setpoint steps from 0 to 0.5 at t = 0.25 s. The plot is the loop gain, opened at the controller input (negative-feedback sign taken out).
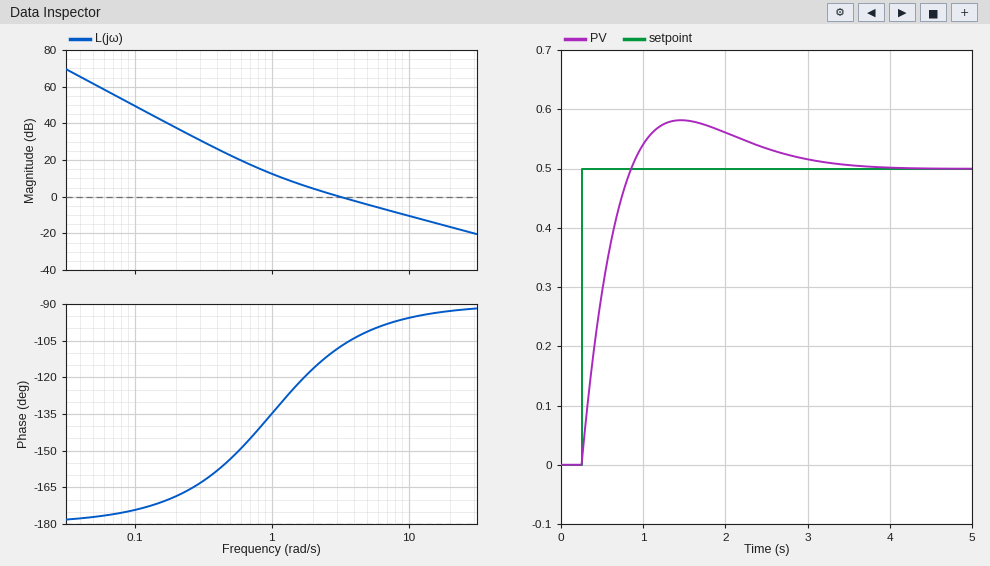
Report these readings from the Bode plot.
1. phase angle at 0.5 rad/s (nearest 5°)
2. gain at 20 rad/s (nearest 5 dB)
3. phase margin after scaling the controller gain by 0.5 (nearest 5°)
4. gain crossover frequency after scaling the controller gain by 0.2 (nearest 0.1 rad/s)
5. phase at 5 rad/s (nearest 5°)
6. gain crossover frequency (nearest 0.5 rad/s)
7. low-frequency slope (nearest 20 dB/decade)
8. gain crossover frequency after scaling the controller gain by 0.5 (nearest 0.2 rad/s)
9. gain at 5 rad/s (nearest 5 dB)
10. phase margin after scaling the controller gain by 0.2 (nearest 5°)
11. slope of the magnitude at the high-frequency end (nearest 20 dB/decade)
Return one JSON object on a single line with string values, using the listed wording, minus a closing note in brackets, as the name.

{"phase angle at 0.5 rad/s": "-155°", "gain at 20 rad/s": "-15 dB", "phase margin after scaling the controller gain by 0.5": "60°", "gain crossover frequency after scaling the controller gain by 0.2": "0.9 rad/s", "phase at 5 rad/s": "-100°", "gain crossover frequency": "3.0 rad/s", "low-frequency slope": "-40 dB/decade", "gain crossover frequency after scaling the controller gain by 0.5": "1.8 rad/s", "gain at 5 rad/s": "-5 dB", "phase margin after scaling the controller gain by 0.2": "40°", "slope of the magnitude at the high-frequency end": "-20 dB/decade"}
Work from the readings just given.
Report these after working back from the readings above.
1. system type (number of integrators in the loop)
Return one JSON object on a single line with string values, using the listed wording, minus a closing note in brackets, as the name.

{"system type": "2"}
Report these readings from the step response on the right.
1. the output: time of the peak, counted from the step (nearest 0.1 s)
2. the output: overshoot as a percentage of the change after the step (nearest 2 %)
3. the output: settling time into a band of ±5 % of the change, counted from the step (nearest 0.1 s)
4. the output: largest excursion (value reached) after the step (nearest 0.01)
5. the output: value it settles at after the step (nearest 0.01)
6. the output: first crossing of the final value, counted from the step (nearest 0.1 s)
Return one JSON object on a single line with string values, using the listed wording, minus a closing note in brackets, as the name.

{"the output: time of the peak, counted from the step": "1.2 s", "the output: overshoot as a percentage of the change after the step": "16 %", "the output: settling time into a band of ±5 % of the change, counted from the step": "2.5 s", "the output: largest excursion (value reached) after the step": "0.58", "the output: value it settles at after the step": "0.50", "the output: first crossing of the final value, counted from the step": "0.6 s"}
